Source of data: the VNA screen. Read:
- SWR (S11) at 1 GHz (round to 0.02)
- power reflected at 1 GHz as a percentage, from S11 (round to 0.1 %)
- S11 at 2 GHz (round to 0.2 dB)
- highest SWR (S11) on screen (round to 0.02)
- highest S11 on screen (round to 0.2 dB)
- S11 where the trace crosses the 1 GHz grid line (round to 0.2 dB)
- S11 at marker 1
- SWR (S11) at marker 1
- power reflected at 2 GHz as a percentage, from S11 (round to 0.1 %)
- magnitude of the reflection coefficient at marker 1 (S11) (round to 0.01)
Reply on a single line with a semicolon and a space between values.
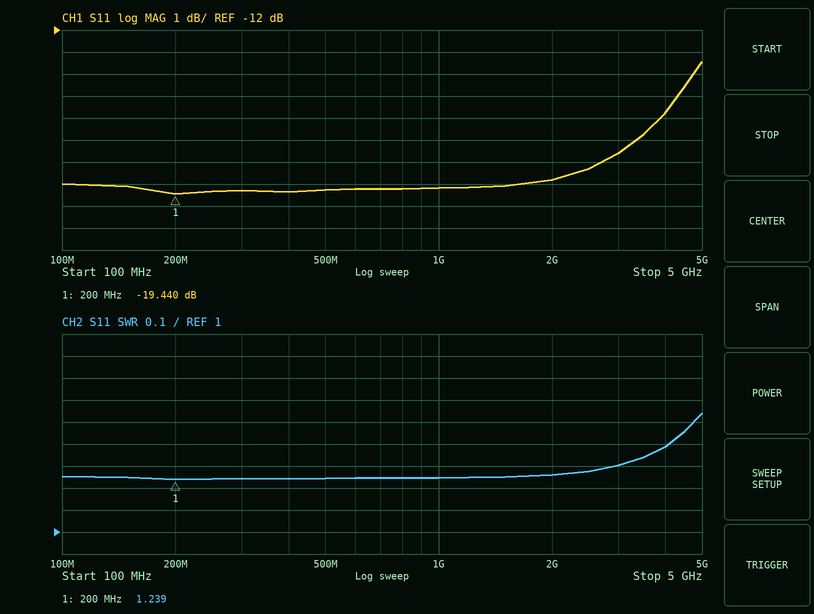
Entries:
1.24; 1.2 %; -18.8 dB; 1.54; -13.4 dB; -19.2 dB; -19.440 dB; 1.239; 1.3 %; 0.11
